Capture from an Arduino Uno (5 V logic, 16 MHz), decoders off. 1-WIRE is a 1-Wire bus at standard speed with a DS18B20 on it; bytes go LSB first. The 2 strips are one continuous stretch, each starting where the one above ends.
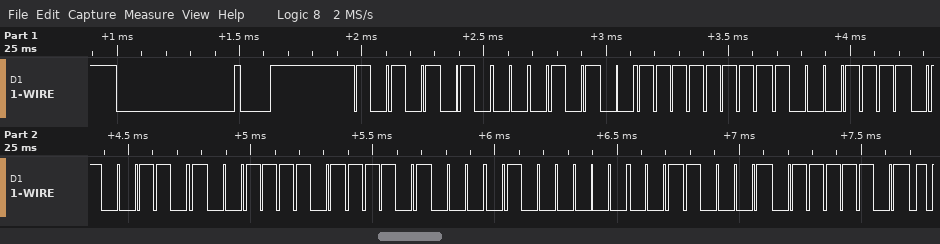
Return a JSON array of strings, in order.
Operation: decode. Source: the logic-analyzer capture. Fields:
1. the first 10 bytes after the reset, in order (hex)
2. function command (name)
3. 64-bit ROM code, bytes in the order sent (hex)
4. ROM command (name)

["55 28 FF F1 B2 BC 17 02 8C BE", "Read Scratchpad", "28 FF F1 B2 BC 17 02 8C", "Match ROM"]
